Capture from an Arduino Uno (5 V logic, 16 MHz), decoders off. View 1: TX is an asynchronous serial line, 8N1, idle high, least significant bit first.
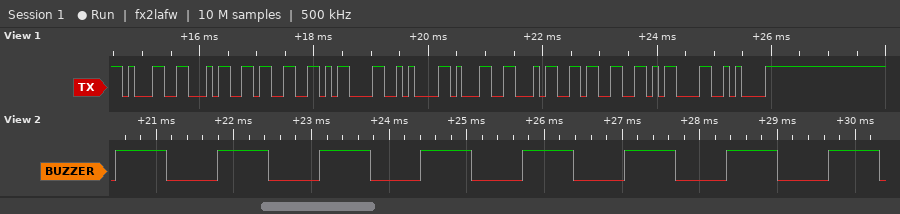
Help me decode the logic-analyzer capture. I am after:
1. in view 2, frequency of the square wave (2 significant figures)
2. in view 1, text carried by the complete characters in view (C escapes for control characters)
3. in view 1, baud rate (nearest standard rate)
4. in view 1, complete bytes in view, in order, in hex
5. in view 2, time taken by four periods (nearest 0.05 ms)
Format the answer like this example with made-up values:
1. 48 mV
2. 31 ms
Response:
1. 760 Hz
2. "143\r\n143\r\n"
3. 9600 baud
4. 31 34 33 0D 0A 31 34 33 0D 0A
5. 5.25 ms
